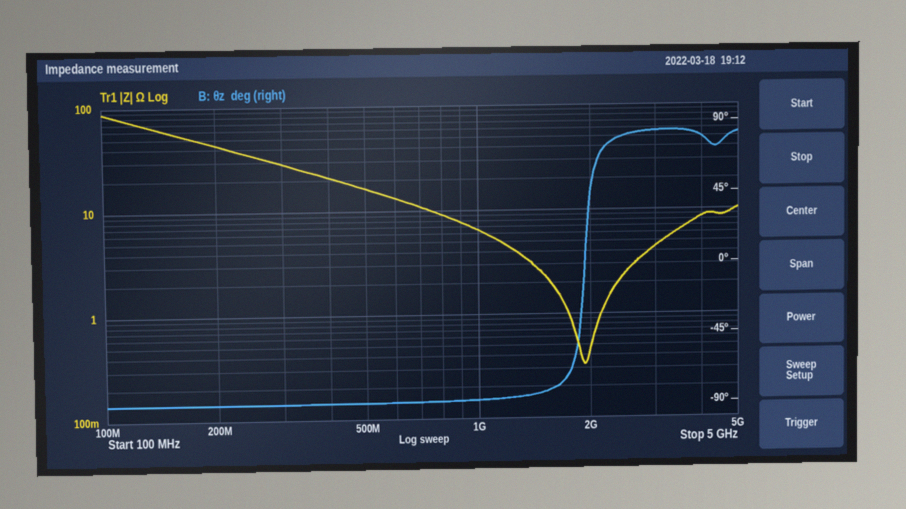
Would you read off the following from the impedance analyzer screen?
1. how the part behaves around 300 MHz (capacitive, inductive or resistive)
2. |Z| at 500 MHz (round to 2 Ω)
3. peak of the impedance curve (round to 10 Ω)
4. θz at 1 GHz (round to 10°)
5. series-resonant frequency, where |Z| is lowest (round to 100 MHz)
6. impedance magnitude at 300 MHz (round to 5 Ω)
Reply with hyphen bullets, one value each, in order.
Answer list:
- capacitive
- 16 Ω
- 90 Ω
- -90°
- 1.9 GHz
- 30 Ω
